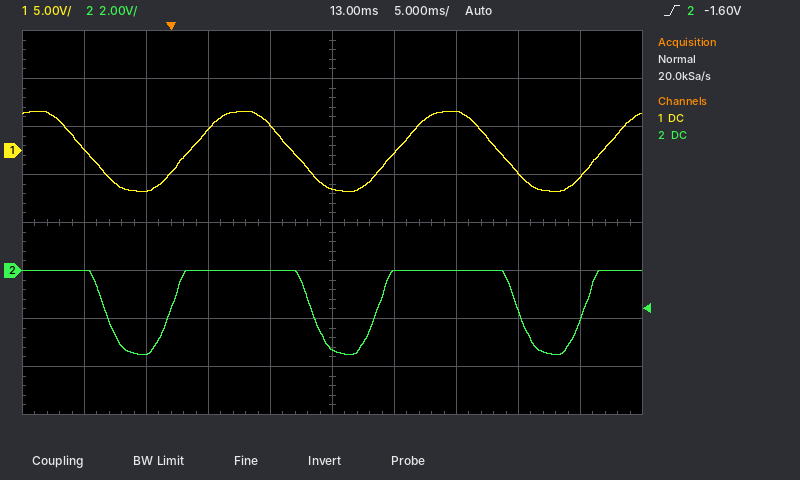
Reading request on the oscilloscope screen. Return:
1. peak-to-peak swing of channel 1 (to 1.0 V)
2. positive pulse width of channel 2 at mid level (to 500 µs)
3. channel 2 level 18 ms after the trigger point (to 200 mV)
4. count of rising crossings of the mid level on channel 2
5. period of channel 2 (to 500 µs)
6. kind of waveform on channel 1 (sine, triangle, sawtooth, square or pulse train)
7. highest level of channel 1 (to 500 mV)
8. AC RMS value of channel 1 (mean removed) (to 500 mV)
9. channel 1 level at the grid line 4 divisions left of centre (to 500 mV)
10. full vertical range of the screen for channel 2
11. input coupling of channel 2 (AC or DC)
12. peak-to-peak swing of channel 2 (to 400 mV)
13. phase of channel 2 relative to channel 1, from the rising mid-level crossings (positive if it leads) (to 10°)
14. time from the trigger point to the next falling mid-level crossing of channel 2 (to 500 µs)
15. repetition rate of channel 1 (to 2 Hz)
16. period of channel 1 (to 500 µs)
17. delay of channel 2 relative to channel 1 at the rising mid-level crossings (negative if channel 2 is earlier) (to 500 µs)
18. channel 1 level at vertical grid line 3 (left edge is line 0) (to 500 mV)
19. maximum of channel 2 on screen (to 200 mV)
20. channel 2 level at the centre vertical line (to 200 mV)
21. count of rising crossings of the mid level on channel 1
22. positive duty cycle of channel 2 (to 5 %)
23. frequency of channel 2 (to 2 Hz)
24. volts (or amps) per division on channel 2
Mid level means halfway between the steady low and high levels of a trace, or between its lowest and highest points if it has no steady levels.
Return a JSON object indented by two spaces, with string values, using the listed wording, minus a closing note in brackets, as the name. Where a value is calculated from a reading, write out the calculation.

{
  "peak-to-peak swing of channel 1": "8.0 V",
  "positive pulse width of channel 2 at mid level": "11.5 ms",
  "channel 2 level 18 ms after the trigger point": "0.0 V",
  "count of rising crossings of the mid level on channel 2": "3",
  "period of channel 2": "16.5 ms",
  "kind of waveform on channel 1": "sine",
  "highest level of channel 1": "4.0 V",
  "AC RMS value of channel 1 (mean removed)": "8.0 V / (2√2) ≈ 2.83 V, so 3.0 V to the nearest 500 mV",
  "channel 1 level at the grid line 4 divisions left of centre": "0.0 V",
  "full vertical range of the screen for channel 2": "16 V",
  "input coupling of channel 2": "DC",
  "peak-to-peak swing of channel 2": "3.6 V",
  "phase of channel 2 relative to channel 1, from the rising mid-level crossings (positive if it leads)": "−360° × (-1.5 ms) / 16.5 ms ≈ +32.7°, so +30° to the nearest 10°",
  "time from the trigger point to the next falling mid-level crossing of channel 2": "11.5 ms",
  "repetition rate of channel 1": "1 / 16.5 ms ≈ 60.6 Hz, so 60 Hz to the nearest 2 Hz",
  "period of channel 1": "16.5 ms",
  "delay of channel 2 relative to channel 1 at the rising mid-level crossings (negative if channel 2 is earlier)": "-1.5 ms",
  "channel 1 level at vertical grid line 3 (left edge is line 0)": "2.0 V",
  "maximum of channel 2 on screen": "0.0 V",
  "channel 2 level at the centre vertical line": "-3.2 V",
  "count of rising crossings of the mid level on channel 1": "3",
  "positive duty cycle of channel 2": "11.5 ms / 16.5 ms ≈ 70 %",
  "frequency of channel 2": "1 / 16.5 ms ≈ 60.6 Hz, so 60 Hz to the nearest 2 Hz",
  "volts (or amps) per division on channel 2": "2 V"
}
